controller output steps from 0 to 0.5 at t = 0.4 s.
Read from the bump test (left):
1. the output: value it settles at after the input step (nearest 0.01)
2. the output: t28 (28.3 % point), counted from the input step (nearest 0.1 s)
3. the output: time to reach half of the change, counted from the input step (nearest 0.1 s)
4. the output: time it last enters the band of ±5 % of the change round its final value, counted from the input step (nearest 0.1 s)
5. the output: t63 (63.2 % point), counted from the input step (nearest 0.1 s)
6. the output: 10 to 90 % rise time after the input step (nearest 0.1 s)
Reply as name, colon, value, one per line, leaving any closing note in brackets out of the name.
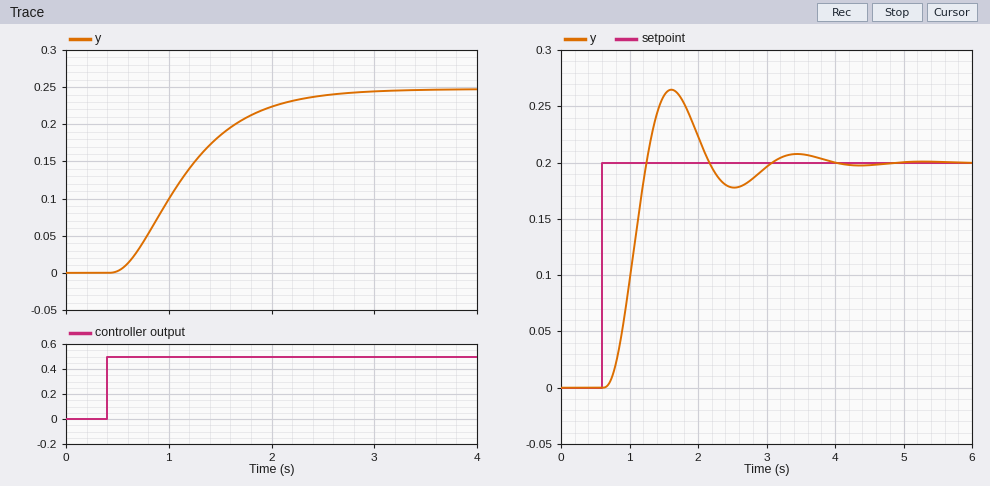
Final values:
the output: value it settles at after the input step: 0.25
the output: t28 (28.3 % point), counted from the input step: 0.5 s
the output: time to reach half of the change, counted from the input step: 0.7 s
the output: time it last enters the band of ±5 % of the change round its final value, counted from the input step: 1.9 s
the output: t63 (63.2 % point), counted from the input step: 0.9 s
the output: 10 to 90 % rise time after the input step: 1.3 s
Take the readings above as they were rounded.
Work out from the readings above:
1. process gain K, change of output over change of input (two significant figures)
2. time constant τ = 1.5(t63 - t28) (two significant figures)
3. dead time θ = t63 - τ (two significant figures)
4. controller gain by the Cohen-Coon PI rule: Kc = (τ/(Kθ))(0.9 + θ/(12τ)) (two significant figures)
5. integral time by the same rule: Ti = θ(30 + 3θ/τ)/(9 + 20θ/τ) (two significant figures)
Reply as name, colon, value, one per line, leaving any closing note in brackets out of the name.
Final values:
process gain K, change of output over change of input: 0.50
time constant τ = 1.5(t63 - t28): 0.60 s
dead time θ = t63 - τ: 0.30 s
controller gain by the Cohen-Coon PI rule: Kc = (τ/(Kθ))(0.9 + θ/(12τ)): 3.8
integral time by the same rule: Ti = θ(30 + 3θ/τ)/(9 + 20θ/τ): 0.50 s
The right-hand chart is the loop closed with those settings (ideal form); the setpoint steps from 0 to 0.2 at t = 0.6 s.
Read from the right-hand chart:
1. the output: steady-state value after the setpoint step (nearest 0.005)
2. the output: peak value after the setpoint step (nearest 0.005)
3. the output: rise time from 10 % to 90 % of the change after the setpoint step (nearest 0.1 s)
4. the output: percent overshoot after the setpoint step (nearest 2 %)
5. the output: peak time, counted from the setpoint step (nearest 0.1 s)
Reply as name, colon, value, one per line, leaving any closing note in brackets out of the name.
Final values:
the output: steady-state value after the setpoint step: 0.200
the output: peak value after the setpoint step: 0.265
the output: rise time from 10 % to 90 % of the change after the setpoint step: 0.4 s
the output: percent overshoot after the setpoint step: 32 %
the output: peak time, counted from the setpoint step: 1.0 s
